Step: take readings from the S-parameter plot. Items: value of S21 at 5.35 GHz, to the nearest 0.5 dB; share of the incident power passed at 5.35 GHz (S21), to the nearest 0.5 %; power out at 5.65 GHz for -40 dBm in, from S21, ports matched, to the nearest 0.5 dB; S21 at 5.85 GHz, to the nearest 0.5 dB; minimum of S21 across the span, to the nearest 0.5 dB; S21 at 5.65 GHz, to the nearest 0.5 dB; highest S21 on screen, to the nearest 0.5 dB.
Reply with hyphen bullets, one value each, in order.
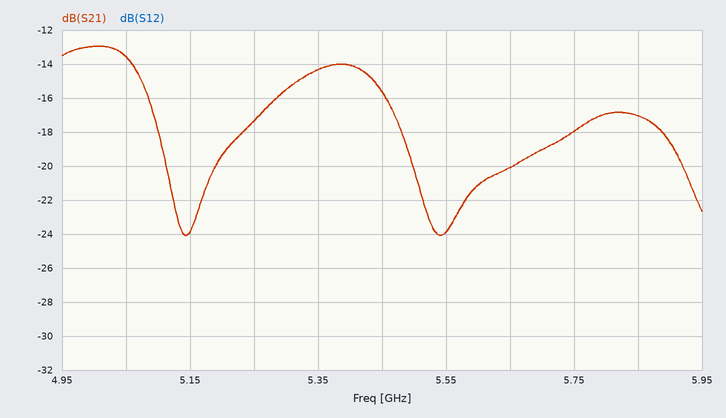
- -14.5 dB
- 3.5 %
- -60.0 dBm
- -17.0 dB
- -24.0 dB
- -20.0 dB
- -13.0 dB
